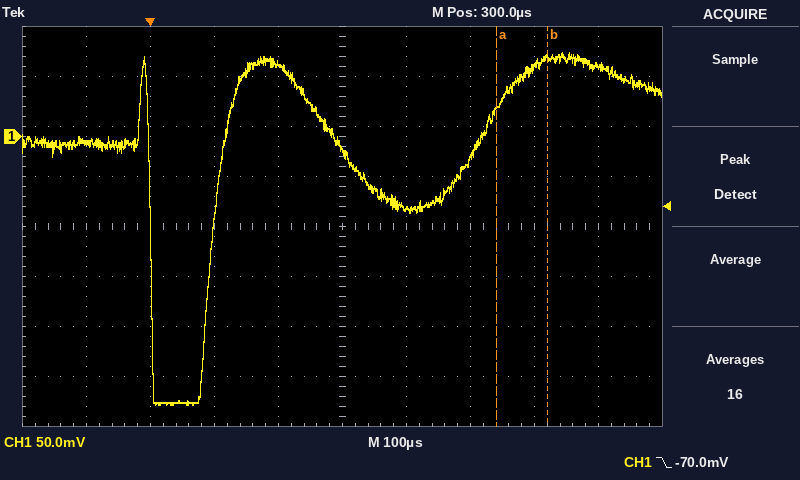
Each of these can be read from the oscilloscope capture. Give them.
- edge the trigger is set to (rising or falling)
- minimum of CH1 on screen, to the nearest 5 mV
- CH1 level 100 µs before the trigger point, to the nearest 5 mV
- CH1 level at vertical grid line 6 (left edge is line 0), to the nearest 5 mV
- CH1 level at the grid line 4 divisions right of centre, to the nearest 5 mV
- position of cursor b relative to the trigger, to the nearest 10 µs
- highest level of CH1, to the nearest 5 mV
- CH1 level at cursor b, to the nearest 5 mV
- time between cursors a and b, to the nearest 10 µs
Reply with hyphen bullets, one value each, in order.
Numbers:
- falling
- -270 mV
- -5 mV
- -70 mV
- 70 mV
- +620 µs
- 85 mV
- 80 mV
- 80 µs
